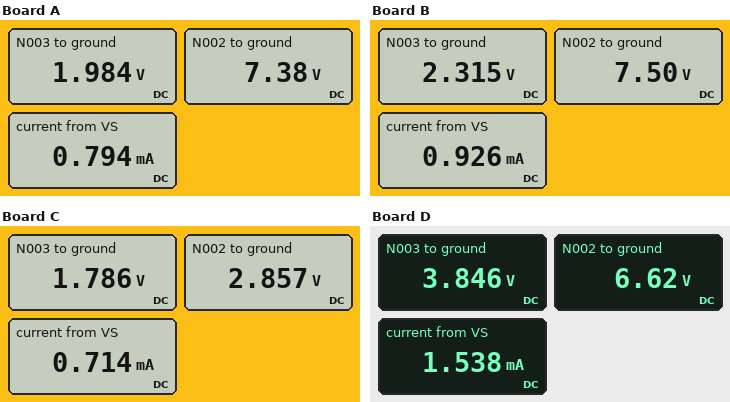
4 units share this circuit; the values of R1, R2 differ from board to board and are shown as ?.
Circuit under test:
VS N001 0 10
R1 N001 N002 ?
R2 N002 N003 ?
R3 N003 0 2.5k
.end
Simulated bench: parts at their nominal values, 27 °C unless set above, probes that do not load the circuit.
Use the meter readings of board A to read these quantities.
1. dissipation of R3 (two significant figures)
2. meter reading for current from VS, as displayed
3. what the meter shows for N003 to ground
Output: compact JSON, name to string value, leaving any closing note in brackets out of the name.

{"dissipation of R3": "1.6 mW", "meter reading for current from VS, as displayed": "0.794 mA", "what the meter shows for N003 to ground": "1.984 V"}
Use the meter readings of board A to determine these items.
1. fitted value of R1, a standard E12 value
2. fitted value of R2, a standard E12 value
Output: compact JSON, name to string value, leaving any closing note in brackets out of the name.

{"fitted value of R1, a standard E12 value": "3.3 kΩ", "fitted value of R2, a standard E12 value": "6.8 kΩ"}
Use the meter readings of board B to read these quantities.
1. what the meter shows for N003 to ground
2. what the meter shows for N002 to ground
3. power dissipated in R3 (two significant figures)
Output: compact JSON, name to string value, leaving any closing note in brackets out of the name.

{"what the meter shows for N003 to ground": "2.315 V", "what the meter shows for N002 to ground": "7.50 V", "power dissipated in R3": "2.1 mW"}
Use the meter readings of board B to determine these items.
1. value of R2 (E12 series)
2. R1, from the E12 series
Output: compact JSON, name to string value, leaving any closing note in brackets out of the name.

{"value of R2": "5.6 kΩ", "R1, from the E12 series": "2.7 kΩ"}
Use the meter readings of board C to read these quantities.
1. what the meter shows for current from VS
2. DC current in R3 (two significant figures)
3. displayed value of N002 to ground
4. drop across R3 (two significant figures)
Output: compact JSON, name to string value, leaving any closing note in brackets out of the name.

{"what the meter shows for current from VS": "0.714 mA", "DC current in R3": "710 µA", "displayed value of N002 to ground": "2.857 V", "drop across R3": "1.8 V"}
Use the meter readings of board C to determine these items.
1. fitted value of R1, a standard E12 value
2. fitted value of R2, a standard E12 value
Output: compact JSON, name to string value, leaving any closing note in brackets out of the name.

{"fitted value of R1, a standard E12 value": "10 kΩ", "fitted value of R2, a standard E12 value": "1.5 kΩ"}
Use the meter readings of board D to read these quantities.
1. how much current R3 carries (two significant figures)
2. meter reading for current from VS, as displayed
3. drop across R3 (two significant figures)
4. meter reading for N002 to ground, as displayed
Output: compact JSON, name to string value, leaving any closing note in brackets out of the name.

{"how much current R3 carries": "1.5 mA", "meter reading for current from VS, as displayed": "1.538 mA", "drop across R3": "3.8 V", "meter reading for N002 to ground, as displayed": "6.62 V"}
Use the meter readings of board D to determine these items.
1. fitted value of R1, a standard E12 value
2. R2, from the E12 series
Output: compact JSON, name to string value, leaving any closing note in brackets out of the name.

{"fitted value of R1, a standard E12 value": "2.2 kΩ", "R2, from the E12 series": "1.8 kΩ"}
